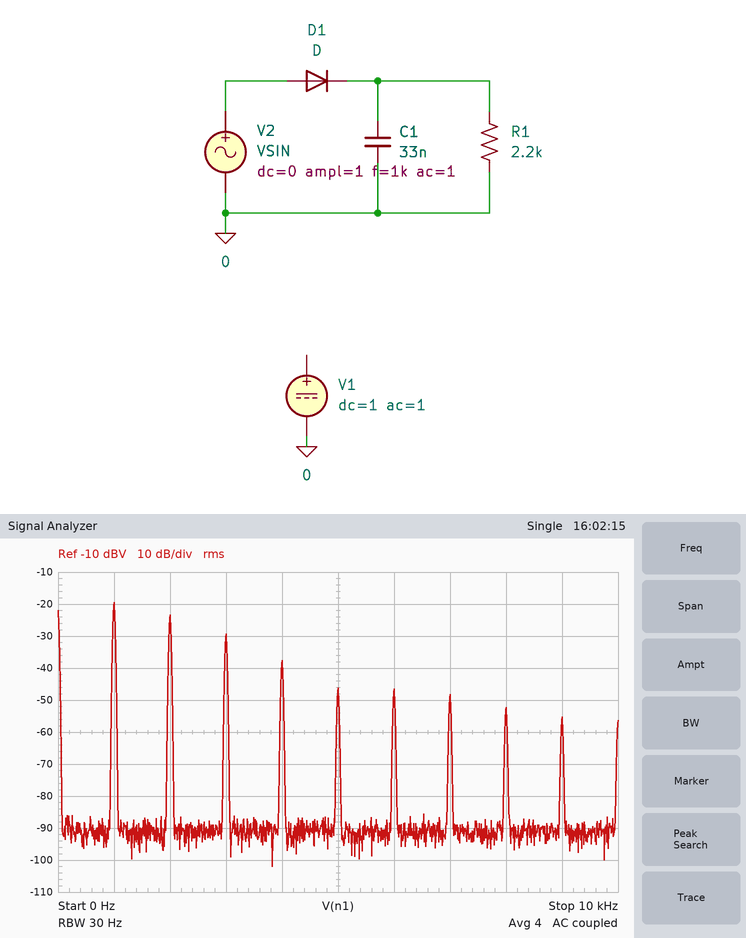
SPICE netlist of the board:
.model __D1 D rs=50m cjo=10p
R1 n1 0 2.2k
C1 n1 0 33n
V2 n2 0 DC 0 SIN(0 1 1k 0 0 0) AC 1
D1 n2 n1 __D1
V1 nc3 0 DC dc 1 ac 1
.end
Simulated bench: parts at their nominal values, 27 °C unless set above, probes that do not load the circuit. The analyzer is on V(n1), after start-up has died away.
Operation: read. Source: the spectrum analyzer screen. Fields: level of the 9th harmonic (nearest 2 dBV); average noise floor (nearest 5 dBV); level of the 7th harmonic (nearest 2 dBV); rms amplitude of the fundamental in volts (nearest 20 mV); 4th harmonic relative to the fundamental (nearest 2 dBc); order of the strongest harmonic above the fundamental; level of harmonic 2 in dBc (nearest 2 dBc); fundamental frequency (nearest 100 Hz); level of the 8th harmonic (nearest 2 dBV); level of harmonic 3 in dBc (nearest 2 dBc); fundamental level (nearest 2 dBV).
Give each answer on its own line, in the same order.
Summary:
-56 dBV
-90 dBV
-48 dBV
100 mV
-18 dBc
2
-4 dBc
1.0 kHz
-52 dBV
-10 dBc
-20 dBV
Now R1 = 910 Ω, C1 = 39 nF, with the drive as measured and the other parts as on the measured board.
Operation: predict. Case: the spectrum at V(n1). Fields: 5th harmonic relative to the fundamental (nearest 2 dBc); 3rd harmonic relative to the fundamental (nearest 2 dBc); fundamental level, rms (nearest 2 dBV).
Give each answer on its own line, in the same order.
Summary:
-30 dBc
-8 dBc
-20 dBV
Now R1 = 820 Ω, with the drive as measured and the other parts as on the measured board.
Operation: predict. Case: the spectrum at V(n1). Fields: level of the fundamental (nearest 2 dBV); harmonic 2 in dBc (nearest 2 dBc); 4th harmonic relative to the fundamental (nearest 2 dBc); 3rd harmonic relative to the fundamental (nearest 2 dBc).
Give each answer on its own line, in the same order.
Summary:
-20 dBV
-2 dBc
-16 dBc
-8 dBc
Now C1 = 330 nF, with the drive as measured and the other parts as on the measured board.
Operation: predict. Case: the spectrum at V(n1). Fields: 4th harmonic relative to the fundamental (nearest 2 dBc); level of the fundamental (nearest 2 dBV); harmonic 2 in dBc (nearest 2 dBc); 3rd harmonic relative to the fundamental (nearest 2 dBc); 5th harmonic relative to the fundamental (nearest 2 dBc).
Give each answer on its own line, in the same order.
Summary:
-16 dBc
-24 dBV
-6 dBc
-12 dBc
-20 dBc
